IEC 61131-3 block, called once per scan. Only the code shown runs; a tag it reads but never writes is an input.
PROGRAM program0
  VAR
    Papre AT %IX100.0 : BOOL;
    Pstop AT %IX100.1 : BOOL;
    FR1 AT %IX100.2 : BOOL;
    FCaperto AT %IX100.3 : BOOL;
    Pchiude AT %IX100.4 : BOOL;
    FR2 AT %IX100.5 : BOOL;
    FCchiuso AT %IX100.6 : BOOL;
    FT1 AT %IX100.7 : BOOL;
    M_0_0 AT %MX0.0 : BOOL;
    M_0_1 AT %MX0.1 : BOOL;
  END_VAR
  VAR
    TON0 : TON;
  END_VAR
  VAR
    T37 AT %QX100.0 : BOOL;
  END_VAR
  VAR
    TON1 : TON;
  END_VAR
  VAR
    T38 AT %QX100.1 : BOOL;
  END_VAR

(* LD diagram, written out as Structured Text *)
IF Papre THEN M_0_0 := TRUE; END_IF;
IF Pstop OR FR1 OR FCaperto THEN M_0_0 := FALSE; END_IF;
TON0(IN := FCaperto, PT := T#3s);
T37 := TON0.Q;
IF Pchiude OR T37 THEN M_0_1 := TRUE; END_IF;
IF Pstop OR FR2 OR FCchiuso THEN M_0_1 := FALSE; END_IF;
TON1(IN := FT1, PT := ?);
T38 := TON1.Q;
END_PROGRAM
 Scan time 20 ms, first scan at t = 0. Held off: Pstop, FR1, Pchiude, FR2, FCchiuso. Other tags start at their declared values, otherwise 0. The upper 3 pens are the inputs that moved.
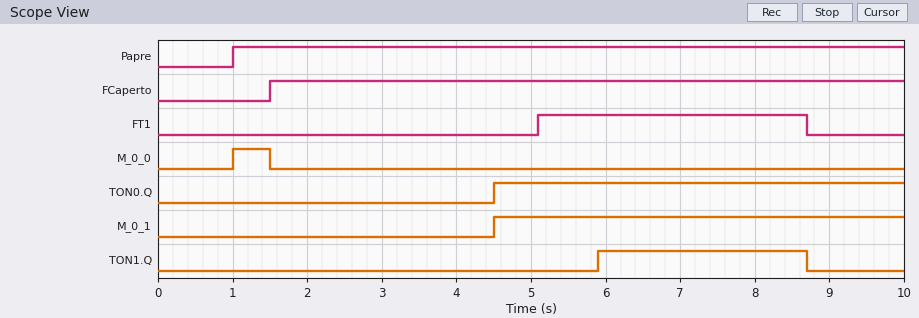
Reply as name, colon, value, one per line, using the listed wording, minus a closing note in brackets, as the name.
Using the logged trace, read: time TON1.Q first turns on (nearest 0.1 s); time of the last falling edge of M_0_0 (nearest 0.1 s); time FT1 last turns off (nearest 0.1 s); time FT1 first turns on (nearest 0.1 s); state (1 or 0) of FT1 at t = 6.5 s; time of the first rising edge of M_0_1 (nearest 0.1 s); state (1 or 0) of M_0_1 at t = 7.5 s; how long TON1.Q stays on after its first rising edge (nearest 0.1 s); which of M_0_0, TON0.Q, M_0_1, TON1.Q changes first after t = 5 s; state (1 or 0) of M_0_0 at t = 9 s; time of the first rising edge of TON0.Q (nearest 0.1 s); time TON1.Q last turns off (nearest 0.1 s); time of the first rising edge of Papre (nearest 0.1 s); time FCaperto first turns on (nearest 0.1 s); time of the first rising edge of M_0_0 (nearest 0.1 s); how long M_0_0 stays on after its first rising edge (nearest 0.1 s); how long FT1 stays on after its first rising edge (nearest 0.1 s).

time TON1.Q first turns on: 5.9 s
time of the last falling edge of M_0_0: 1.5 s
time FT1 last turns off: 8.7 s
time FT1 first turns on: 5.1 s
state (1 or 0) of FT1 at t = 6.5 s: 1
time of the first rising edge of M_0_1: 4.5 s
state (1 or 0) of M_0_1 at t = 7.5 s: 1
how long TON1.Q stays on after its first rising edge: 2.8 s
which of M_0_0, TON0.Q, M_0_1, TON1.Q changes first after t = 5 s: TON1.Q
state (1 or 0) of M_0_0 at t = 9 s: 0
time of the first rising edge of TON0.Q: 4.5 s
time TON1.Q last turns off: 8.7 s
time of the first rising edge of Papre: 1.0 s
time FCaperto first turns on: 1.5 s
time of the first rising edge of M_0_0: 1.0 s
how long M_0_0 stays on after its first rising edge: 0.5 s
how long FT1 stays on after its first rising edge: 3.6 s
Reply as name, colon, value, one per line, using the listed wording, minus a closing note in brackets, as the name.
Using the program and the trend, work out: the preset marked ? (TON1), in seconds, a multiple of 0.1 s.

the preset marked ? (TON1), in seconds, a multiple of 0.1 s: 0.8 s
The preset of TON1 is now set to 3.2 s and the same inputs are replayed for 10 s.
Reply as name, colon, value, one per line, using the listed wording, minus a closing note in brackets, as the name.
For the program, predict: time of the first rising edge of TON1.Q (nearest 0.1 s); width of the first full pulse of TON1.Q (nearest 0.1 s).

time of the first rising edge of TON1.Q: 8.3 s
width of the first full pulse of TON1.Q: 0.4 s
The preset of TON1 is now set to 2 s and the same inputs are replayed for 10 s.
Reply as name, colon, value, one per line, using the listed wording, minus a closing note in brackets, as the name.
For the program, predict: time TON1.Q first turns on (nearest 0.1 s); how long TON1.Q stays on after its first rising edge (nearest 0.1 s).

time TON1.Q first turns on: 7.1 s
how long TON1.Q stays on after its first rising edge: 1.6 s
